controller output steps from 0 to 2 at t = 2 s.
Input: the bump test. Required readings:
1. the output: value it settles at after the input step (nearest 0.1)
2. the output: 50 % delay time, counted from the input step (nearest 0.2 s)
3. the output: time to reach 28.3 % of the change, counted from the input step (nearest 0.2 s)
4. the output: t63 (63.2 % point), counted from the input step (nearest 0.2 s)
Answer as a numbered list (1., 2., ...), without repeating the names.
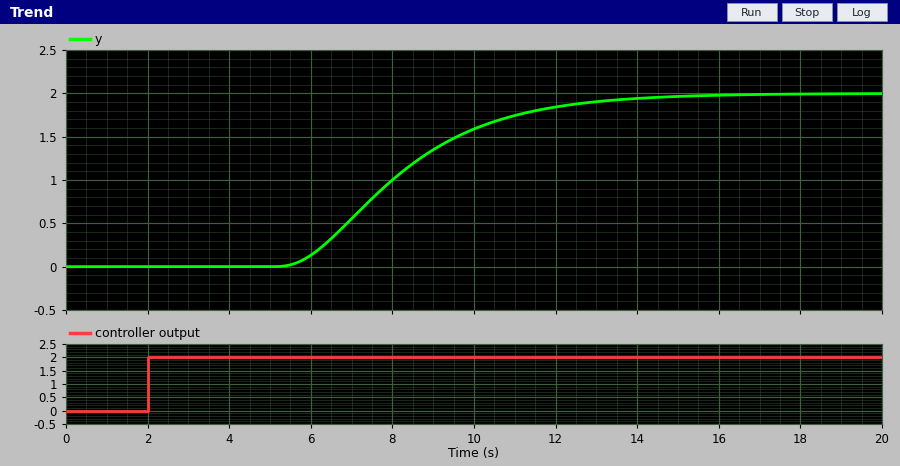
1. 2.0
2. 6.0 s
3. 5.0 s
4. 6.8 s
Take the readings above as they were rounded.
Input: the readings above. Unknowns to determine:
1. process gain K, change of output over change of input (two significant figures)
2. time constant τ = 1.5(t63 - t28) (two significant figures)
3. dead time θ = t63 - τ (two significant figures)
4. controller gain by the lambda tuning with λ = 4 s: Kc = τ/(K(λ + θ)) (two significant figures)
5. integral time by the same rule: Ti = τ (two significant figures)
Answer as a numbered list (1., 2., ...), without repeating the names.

1. 1.0
2. 2.7 s
3. 4.1 s
4. 0.33
5. 2.7 s
